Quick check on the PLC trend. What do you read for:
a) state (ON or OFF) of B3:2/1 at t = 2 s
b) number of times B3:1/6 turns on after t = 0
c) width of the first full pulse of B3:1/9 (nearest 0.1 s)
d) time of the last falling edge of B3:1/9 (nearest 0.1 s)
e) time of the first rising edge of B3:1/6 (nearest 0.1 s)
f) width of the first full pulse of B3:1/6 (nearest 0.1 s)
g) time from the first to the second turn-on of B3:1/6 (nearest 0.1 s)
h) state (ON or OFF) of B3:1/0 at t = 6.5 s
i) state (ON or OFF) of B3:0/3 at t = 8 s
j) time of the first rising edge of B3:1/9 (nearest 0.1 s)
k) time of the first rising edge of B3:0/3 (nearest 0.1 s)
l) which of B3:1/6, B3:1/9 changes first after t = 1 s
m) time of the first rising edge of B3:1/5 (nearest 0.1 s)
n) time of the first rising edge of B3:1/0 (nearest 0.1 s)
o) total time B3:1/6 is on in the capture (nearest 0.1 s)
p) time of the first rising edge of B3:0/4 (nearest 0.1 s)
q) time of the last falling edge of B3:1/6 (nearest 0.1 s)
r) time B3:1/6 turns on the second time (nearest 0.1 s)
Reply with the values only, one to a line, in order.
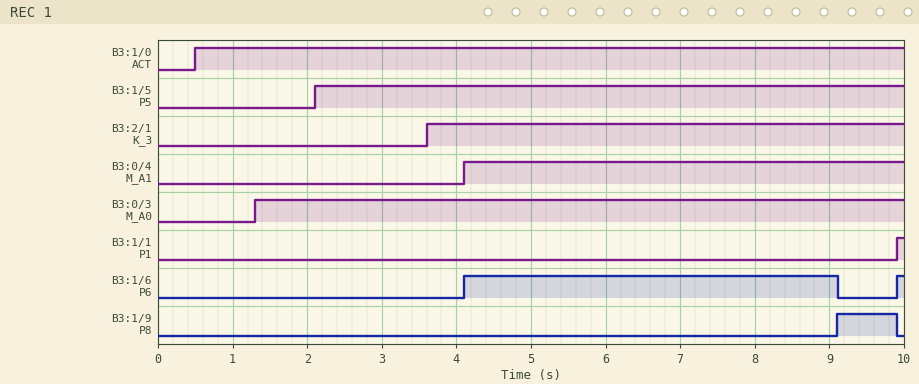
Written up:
OFF
2
0.8 s
9.9 s
4.1 s
5.0 s
5.8 s
ON
ON
9.1 s
1.3 s
B3:1/6
2.1 s
0.5 s
5.1 s
4.1 s
9.1 s
9.9 s
